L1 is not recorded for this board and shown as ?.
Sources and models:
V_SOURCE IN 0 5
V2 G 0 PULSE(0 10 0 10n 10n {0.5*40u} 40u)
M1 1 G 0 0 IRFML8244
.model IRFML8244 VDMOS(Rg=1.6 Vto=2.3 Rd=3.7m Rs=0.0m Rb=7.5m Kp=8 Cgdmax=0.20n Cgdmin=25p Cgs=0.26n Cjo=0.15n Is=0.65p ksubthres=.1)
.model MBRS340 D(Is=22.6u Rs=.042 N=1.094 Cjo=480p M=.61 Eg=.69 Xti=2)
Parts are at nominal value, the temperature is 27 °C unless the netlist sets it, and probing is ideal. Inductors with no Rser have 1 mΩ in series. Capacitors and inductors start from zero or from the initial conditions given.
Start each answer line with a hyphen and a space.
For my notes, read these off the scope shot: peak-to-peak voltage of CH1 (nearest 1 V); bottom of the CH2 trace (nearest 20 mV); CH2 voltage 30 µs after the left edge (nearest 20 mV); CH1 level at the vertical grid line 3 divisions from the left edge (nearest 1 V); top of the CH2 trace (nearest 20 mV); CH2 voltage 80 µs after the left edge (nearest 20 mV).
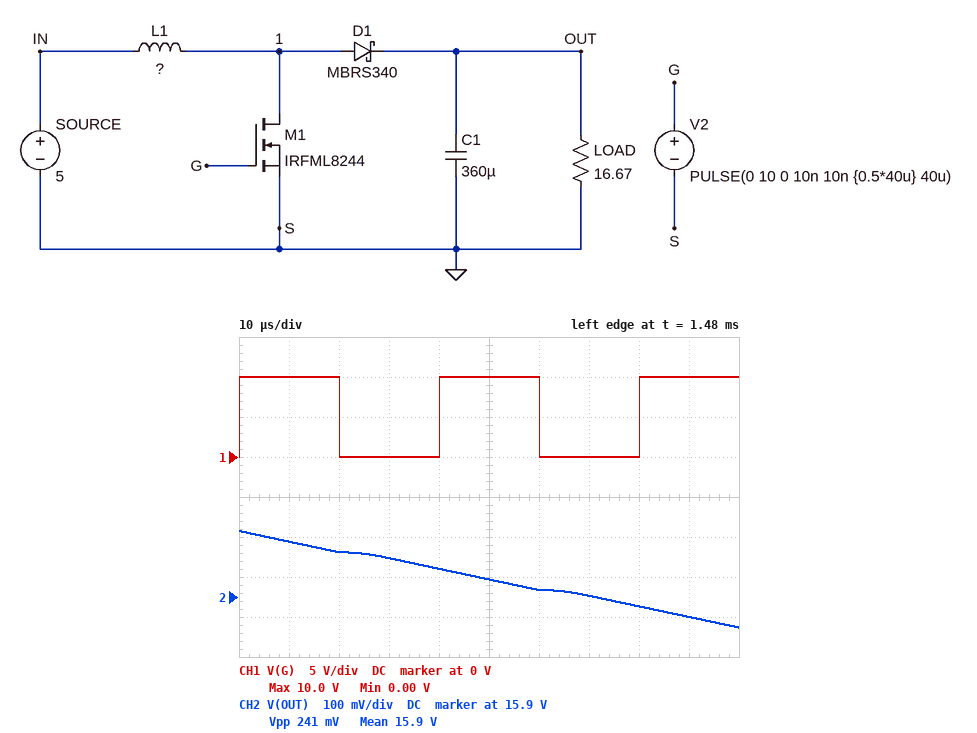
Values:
- 10 V
- 15.82 V
- 16.00 V
- 0 V
- 16.06 V
- 15.88 V
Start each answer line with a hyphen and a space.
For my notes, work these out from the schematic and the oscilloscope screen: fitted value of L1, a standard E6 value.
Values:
- 100 µH
